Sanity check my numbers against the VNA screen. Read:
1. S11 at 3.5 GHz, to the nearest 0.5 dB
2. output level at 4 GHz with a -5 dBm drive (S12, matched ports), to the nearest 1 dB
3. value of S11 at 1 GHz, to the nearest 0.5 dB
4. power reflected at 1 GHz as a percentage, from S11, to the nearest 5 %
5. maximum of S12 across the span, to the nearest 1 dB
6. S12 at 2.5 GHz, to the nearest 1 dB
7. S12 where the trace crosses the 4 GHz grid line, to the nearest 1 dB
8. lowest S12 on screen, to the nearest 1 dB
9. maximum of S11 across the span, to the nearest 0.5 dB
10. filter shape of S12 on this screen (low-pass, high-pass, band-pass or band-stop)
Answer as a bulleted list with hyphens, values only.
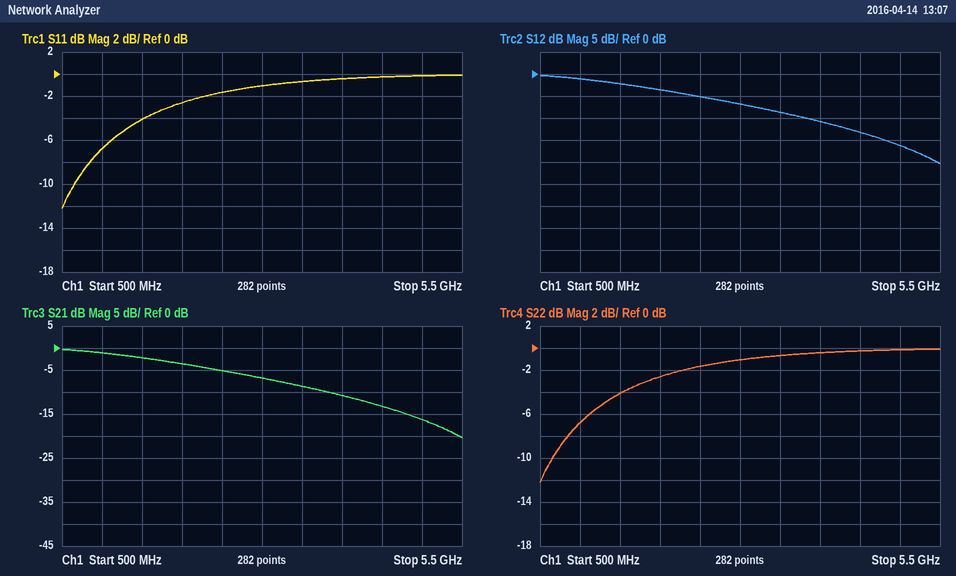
- -0.5 dB
- -16 dBm
- -7.0 dB
- 20 %
- 0 dB
- -5 dB
- -11 dB
- -20 dB
- 0.0 dB
- low-pass
